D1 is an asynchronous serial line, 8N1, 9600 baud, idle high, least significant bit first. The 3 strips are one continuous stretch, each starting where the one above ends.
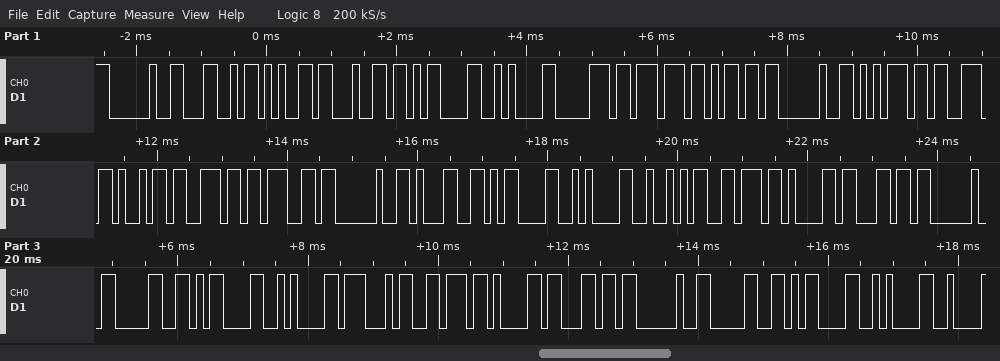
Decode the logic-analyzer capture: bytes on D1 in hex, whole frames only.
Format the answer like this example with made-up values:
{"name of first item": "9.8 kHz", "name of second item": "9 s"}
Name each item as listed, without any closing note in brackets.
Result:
{"bytes on D1 in hex, whole frames only": "20 4C 65 64 0D 0A 70 77 6D 20 75 73 69 6E 67 20 31 0D 0A 52 76 61 6C 20 30 0D 0A 47 76 61 6C 20 30 0D 0A"}
